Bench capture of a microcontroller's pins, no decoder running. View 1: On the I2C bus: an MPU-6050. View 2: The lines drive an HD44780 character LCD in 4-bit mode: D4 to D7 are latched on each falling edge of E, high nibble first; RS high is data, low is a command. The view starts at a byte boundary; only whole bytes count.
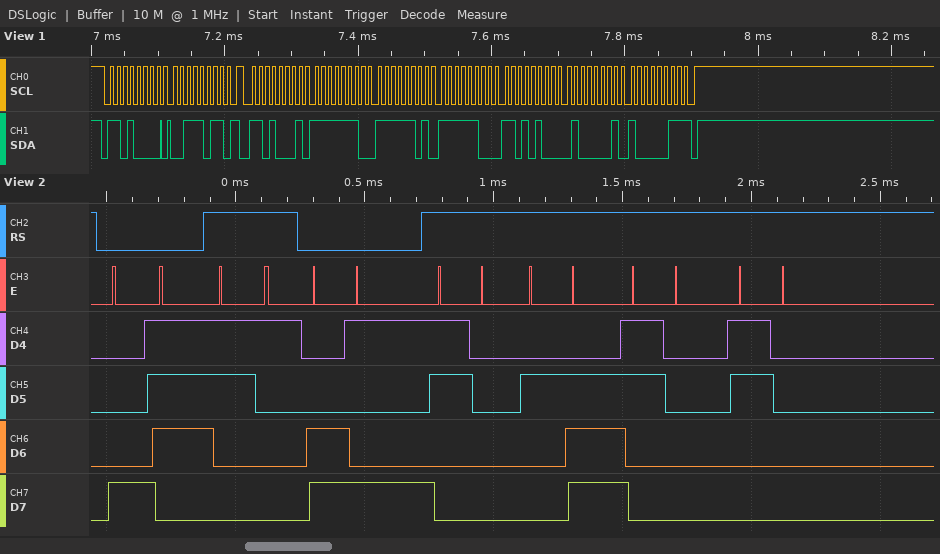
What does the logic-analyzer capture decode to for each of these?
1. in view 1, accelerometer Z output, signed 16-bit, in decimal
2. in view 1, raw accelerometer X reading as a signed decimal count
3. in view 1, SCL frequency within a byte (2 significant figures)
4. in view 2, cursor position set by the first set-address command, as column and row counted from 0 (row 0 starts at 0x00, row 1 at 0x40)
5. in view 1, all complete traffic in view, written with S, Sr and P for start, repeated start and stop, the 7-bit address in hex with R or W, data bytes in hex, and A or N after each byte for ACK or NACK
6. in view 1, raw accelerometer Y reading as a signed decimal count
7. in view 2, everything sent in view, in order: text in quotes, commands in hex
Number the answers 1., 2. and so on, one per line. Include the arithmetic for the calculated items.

1. 0x4183 = 16771
2. 0xFEFD = -259
3. 100 kHz
4. column 7, row 0
5. S 68W A 3B A Sr 68R A FE A FD A FC A D4 A 41 A 83 N P
6. 0xFCD4 = -812
7. 0x87 "1" 0xC9 "0.00"
